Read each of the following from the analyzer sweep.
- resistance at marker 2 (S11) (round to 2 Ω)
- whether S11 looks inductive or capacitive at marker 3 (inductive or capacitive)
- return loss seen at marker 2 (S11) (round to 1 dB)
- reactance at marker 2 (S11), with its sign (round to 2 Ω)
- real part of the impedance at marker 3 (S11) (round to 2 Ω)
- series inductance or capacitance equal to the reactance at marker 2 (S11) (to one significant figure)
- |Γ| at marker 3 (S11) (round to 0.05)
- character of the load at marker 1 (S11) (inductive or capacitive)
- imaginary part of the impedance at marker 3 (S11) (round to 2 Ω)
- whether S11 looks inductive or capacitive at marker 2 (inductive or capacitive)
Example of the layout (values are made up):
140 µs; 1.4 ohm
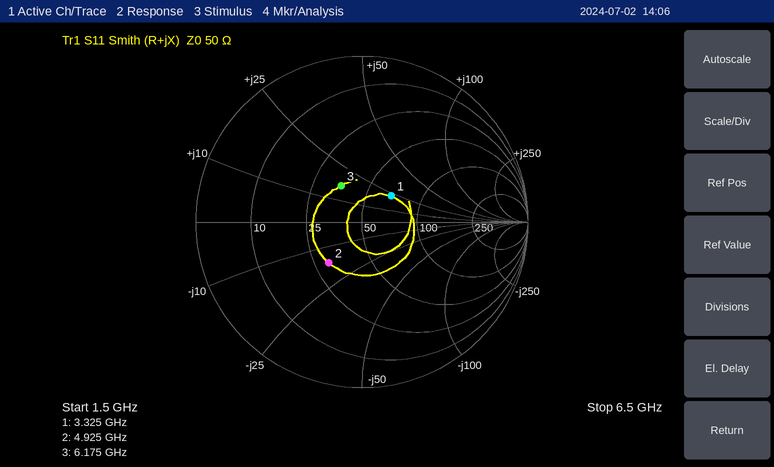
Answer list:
30 Ω; inductive; 10 dB; -16 Ω; 36 Ω; 2 pF; 0.25; inductive; +16 Ω; capacitive
